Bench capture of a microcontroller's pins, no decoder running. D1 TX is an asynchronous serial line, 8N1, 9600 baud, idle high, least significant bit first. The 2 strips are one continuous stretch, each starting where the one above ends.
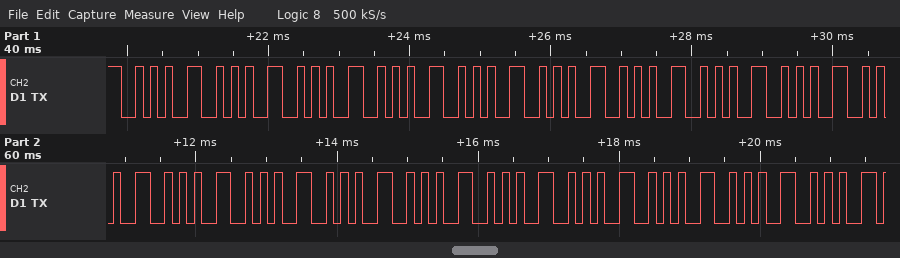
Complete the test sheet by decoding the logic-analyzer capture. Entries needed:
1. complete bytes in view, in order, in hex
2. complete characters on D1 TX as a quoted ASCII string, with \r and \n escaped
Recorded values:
0x2A 0x2A 0x2A 0x2A 0x2A 0x2A 0x2A 0x2A 0x2A 0x2A 0x2A 0x2A 0x2A 0x2A 0x2A 0x2A 0x2A 0x2A 0x2A
"*******************"
